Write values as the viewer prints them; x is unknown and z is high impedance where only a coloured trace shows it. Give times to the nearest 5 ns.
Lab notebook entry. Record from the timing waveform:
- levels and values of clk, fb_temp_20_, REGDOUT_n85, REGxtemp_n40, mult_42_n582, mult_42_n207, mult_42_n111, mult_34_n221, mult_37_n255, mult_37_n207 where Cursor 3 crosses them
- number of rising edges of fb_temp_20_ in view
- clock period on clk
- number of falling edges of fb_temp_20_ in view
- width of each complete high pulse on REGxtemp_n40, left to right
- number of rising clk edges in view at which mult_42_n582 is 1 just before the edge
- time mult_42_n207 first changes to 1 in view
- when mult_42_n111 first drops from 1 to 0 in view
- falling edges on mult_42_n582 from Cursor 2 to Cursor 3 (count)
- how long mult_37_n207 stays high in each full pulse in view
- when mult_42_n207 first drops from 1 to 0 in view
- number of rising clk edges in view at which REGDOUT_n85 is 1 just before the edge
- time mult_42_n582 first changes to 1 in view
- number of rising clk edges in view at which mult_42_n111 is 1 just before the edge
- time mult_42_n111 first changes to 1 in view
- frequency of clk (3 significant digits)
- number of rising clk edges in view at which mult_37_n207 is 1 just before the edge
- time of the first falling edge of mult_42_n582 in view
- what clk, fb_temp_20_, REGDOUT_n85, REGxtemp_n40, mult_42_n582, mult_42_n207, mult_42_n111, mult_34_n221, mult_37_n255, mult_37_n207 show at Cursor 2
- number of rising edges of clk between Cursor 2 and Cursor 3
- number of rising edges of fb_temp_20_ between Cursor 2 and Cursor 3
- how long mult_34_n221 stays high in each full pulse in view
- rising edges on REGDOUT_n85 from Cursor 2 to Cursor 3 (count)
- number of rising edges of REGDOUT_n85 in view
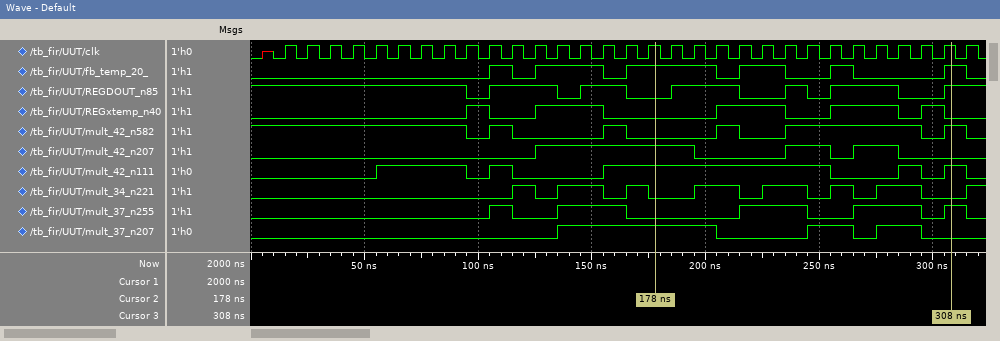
clk=1, fb_temp_20_=1, REGDOUT_n85=1, REGxtemp_n40=0, mult_42_n582=1, mult_42_n207=0, mult_42_n111=1, mult_34_n221=0, mult_37_n255=1, mult_37_n207=0
6
10 ns
6
10 ns, 30 ns, 30 ns, 30 ns, 10 ns
19
125 ns
95 ns
2
70 ns, 20 ns, 20 ns
195 ns
22
105 ns
17
55 ns
100 MHz
11
95 ns
clk=1, fb_temp_20_=1, REGDOUT_n85=0, REGxtemp_n40=0, mult_42_n582=0, mult_42_n207=1, mult_42_n111=1, mult_34_n221=0, mult_37_n255=0, mult_37_n207=1
13
3
10 ns, 20 ns, 10 ns, 20 ns, 20 ns, 10 ns, 20 ns
4
6
